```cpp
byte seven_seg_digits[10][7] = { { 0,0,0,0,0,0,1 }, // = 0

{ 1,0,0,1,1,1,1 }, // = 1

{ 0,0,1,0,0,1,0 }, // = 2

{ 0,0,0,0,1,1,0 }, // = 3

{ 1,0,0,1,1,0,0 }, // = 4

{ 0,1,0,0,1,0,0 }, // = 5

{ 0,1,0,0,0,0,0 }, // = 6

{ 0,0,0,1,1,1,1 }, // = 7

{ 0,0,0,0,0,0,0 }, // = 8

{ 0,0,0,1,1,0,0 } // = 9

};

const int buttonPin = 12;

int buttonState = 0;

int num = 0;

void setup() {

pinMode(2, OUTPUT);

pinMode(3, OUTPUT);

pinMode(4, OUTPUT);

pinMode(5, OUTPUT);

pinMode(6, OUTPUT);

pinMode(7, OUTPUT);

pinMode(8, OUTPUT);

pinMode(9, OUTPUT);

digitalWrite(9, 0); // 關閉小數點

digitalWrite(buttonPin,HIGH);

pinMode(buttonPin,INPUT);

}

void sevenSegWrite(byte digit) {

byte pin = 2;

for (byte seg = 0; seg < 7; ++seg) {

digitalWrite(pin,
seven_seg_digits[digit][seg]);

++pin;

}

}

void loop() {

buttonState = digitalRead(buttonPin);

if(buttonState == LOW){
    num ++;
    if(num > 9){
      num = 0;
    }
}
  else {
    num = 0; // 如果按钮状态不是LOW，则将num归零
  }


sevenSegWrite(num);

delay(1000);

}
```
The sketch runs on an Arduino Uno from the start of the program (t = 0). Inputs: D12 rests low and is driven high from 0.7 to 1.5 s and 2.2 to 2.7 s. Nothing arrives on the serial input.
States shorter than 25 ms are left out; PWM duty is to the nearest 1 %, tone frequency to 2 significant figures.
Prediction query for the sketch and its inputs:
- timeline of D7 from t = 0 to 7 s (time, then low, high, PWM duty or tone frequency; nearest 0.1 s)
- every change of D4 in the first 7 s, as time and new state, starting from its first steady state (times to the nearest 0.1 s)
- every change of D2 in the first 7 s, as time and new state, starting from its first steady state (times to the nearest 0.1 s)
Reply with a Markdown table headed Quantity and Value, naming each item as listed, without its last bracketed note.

| Quantity | Value |
|---|---|
| timeline of D7 from t = 0 to 7 s | 0 s high; 1 s low; 2 s high; 5 s low |
| every change of D4 in the first 7 s, as time and new state, starting from its first steady state | 0 s low; 3 s high; 4 s low |
| every change of D2 in the first 7 s, as time and new state, starting from its first steady state | 0 s high; 1 s low; 2 s high; 3 s low; 5 s high; 6 s low |
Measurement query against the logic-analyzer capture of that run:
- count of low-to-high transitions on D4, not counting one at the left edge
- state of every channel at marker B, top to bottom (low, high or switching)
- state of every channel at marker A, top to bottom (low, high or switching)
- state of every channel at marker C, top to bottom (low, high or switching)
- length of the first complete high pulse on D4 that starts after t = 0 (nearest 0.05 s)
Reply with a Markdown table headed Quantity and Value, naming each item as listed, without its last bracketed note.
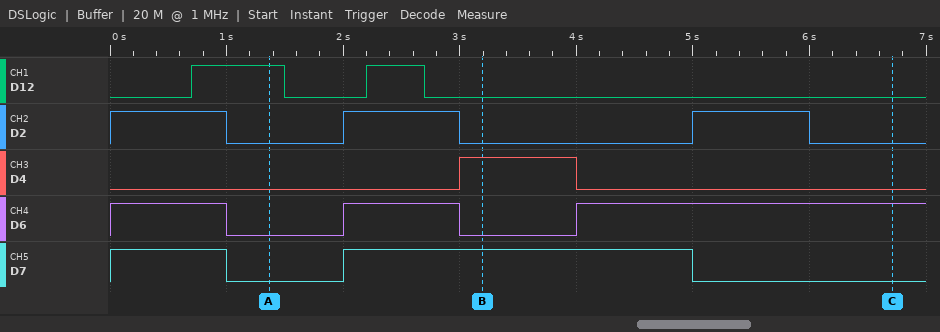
| Quantity | Value |
|---|---|
| count of low-to-high transitions on D4, not counting one at the left edge | 1 |
| state of every channel at marker B, top to bottom | D12 low, D2 low, D4 high, D6 low, D7 high |
| state of every channel at marker A, top to bottom | D12 high, D2 low, D4 low, D6 low, D7 low |
| state of every channel at marker C, top to bottom | D12 low, D2 low, D4 low, D6 high, D7 low |
| length of the first complete high pulse on D4 that starts after t = 0 | 1.00 s |
